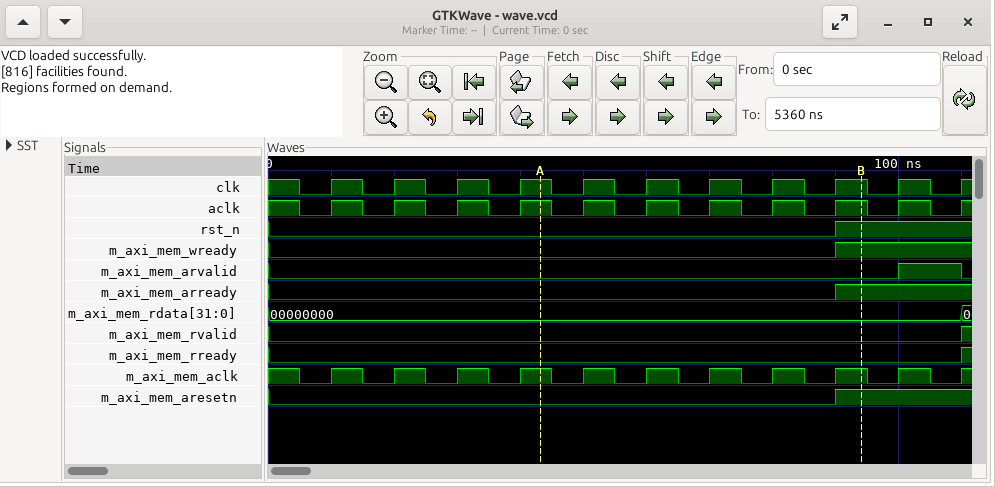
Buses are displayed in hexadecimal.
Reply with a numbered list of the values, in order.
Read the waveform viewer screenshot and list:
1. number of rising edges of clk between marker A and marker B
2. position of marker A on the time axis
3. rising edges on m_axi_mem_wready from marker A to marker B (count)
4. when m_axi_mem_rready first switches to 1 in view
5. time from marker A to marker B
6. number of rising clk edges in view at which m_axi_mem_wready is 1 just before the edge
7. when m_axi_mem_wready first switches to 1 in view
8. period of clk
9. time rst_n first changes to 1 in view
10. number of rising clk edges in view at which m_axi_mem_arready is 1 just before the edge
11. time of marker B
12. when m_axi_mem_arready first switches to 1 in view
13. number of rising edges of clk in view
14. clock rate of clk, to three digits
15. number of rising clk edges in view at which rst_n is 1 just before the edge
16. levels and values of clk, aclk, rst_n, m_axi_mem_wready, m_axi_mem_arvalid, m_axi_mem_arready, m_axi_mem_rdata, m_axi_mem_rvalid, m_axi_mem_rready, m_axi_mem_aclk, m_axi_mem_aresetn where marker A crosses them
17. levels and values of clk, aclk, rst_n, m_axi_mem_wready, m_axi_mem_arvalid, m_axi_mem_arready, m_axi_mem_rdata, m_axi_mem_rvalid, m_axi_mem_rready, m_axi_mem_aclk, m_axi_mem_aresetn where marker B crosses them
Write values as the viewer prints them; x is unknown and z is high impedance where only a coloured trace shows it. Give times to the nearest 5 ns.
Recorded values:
1. 5
2. 45 ns
3. 1
4. 110 ns
5. 50 ns
6. 2
7. 90 ns
8. 10 ns
9. 90 ns
10. 2
11. 95 ns
12. 90 ns
13. 11
14. 100 MHz
15. 2
16. clk=1, aclk=1, rst_n=0, m_axi_mem_wready=0, m_axi_mem_arvalid=0, m_axi_mem_arready=0, m_axi_mem_rdata=00000000, m_axi_mem_rvalid=0, m_axi_mem_rready=0, m_axi_mem_aclk=1, m_axi_mem_aresetn=0
17. clk=1, aclk=1, rst_n=1, m_axi_mem_wready=1, m_axi_mem_arvalid=0, m_axi_mem_arready=1, m_axi_mem_rdata=00000000, m_axi_mem_rvalid=0, m_axi_mem_rready=0, m_axi_mem_aclk=1, m_axi_mem_aresetn=1
